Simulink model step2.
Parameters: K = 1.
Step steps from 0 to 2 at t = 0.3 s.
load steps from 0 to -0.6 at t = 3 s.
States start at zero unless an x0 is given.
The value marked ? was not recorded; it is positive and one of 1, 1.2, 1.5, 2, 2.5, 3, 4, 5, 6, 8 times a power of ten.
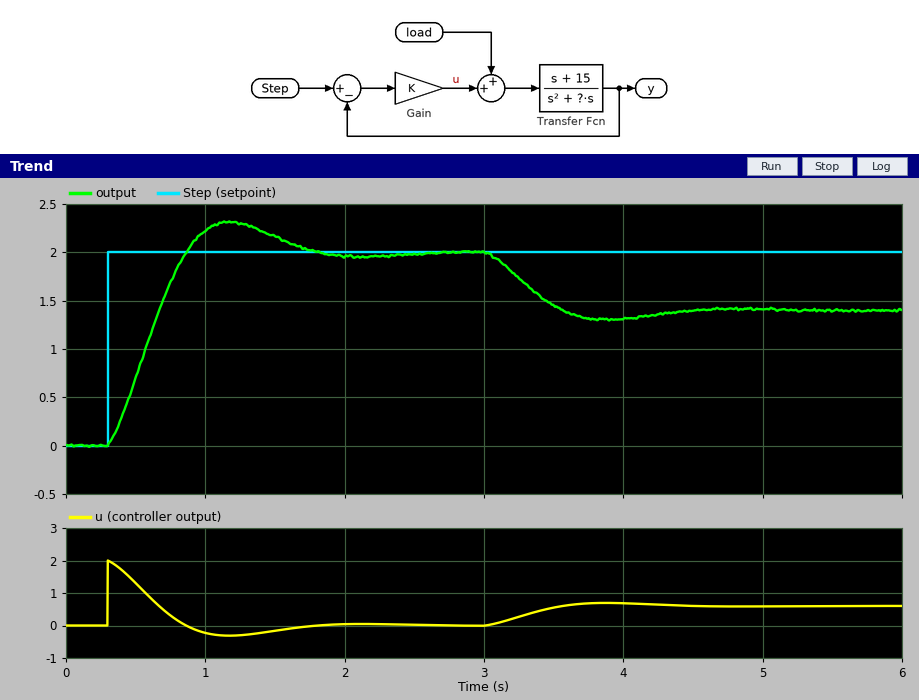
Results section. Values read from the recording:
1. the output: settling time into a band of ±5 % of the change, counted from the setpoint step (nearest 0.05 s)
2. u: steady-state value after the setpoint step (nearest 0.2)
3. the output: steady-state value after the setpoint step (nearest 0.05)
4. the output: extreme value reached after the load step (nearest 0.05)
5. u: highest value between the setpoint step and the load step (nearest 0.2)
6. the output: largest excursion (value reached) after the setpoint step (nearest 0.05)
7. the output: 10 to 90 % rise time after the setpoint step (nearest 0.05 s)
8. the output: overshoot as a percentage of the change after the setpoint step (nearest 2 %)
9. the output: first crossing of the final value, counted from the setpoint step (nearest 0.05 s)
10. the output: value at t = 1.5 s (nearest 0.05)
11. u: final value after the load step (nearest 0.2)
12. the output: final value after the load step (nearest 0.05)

1.30 s
0.0
2.00
1.30
2.0
2.30
0.40 s
16 %
0.55 s
2.15
0.6
1.40
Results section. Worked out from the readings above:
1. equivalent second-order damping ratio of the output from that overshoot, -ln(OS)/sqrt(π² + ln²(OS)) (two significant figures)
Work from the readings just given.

0.50
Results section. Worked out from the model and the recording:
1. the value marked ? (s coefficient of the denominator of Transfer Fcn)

3
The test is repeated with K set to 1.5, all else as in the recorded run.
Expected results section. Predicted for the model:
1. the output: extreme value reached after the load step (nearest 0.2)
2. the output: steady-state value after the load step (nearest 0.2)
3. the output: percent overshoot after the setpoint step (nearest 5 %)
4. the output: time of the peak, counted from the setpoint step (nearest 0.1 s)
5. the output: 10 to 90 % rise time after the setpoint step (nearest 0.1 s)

1.6
1.6
20 %
0.7 s
0.3 s
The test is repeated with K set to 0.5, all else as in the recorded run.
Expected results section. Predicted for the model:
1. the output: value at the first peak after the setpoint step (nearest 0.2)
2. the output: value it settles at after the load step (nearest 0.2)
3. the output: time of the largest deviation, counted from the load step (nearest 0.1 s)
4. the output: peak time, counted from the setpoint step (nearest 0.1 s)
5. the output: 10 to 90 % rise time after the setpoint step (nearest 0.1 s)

2.2
0.8
1.4 s
1.4 s
0.7 s
